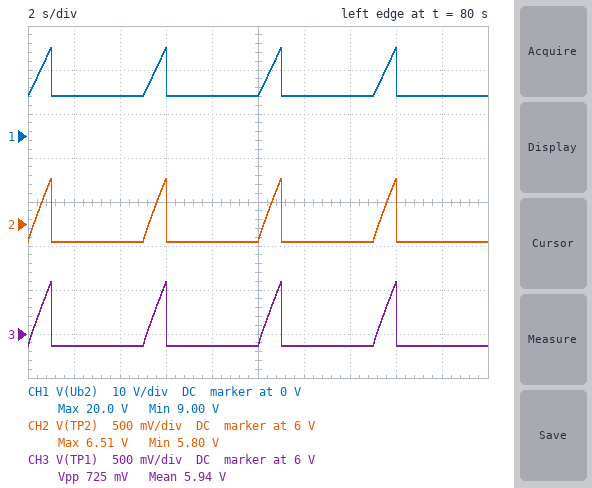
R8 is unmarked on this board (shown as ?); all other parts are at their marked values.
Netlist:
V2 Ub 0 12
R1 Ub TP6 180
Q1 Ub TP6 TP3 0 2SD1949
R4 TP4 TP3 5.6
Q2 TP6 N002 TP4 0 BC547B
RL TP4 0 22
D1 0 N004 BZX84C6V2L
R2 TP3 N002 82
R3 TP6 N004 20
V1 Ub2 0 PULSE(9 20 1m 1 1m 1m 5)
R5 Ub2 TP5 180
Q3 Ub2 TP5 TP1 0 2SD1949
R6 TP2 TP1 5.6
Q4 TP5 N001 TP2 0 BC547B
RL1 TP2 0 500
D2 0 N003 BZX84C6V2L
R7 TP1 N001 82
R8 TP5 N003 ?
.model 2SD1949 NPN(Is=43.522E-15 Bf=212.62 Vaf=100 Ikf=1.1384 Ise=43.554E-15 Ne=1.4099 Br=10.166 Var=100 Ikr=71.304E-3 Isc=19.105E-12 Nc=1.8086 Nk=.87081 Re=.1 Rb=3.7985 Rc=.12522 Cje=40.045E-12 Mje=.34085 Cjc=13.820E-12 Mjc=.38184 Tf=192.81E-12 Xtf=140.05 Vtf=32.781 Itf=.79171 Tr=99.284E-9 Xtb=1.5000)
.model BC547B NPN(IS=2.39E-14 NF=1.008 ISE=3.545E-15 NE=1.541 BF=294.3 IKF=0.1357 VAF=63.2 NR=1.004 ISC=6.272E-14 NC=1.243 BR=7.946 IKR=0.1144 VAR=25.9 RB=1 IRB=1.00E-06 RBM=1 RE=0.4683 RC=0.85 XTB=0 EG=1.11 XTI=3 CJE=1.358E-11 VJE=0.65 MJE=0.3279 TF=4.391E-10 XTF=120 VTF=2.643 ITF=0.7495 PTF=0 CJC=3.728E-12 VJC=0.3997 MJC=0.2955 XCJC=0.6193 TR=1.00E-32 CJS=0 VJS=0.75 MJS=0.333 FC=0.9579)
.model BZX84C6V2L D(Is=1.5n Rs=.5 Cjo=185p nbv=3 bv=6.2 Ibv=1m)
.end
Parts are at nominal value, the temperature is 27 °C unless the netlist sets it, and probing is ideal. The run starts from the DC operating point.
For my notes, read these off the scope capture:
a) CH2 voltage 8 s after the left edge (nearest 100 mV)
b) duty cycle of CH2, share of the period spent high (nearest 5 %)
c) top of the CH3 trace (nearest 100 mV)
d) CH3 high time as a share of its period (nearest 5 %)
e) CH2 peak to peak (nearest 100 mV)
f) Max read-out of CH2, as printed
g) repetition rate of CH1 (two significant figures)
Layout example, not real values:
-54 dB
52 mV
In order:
5.8 V
10 %
6.6 V
10 %
700 mV
6.51 V
200 mHz
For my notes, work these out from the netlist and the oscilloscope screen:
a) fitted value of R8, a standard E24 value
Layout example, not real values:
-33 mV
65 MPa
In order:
10 Ω
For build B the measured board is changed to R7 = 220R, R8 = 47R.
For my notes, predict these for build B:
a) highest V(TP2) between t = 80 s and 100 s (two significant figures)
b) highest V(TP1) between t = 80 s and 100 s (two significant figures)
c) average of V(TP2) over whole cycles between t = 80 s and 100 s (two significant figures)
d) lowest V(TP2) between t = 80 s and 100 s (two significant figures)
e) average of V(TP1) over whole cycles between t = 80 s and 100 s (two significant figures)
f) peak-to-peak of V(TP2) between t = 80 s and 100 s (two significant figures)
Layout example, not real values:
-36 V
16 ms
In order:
8.5 V
8.6 V
6.4 V
6.2 V
6.5 V
2.4 V
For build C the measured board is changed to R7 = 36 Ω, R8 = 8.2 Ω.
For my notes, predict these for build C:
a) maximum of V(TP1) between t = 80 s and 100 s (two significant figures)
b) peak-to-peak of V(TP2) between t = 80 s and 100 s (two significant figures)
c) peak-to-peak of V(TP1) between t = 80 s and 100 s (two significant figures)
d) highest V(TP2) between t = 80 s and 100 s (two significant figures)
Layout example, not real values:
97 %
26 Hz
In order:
6.5 V
620 mV
630 mV
6.4 V
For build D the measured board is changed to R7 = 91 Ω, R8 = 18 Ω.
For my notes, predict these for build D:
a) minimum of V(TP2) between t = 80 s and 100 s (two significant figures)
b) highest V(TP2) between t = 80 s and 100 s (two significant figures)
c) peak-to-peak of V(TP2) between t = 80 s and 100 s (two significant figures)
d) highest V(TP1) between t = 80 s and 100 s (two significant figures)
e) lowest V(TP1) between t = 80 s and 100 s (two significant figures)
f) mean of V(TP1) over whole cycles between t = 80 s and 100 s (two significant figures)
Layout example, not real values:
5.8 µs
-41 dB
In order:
5.9 V
7.0 V
1.1 V
7.1 V
6.0 V
6.1 V
